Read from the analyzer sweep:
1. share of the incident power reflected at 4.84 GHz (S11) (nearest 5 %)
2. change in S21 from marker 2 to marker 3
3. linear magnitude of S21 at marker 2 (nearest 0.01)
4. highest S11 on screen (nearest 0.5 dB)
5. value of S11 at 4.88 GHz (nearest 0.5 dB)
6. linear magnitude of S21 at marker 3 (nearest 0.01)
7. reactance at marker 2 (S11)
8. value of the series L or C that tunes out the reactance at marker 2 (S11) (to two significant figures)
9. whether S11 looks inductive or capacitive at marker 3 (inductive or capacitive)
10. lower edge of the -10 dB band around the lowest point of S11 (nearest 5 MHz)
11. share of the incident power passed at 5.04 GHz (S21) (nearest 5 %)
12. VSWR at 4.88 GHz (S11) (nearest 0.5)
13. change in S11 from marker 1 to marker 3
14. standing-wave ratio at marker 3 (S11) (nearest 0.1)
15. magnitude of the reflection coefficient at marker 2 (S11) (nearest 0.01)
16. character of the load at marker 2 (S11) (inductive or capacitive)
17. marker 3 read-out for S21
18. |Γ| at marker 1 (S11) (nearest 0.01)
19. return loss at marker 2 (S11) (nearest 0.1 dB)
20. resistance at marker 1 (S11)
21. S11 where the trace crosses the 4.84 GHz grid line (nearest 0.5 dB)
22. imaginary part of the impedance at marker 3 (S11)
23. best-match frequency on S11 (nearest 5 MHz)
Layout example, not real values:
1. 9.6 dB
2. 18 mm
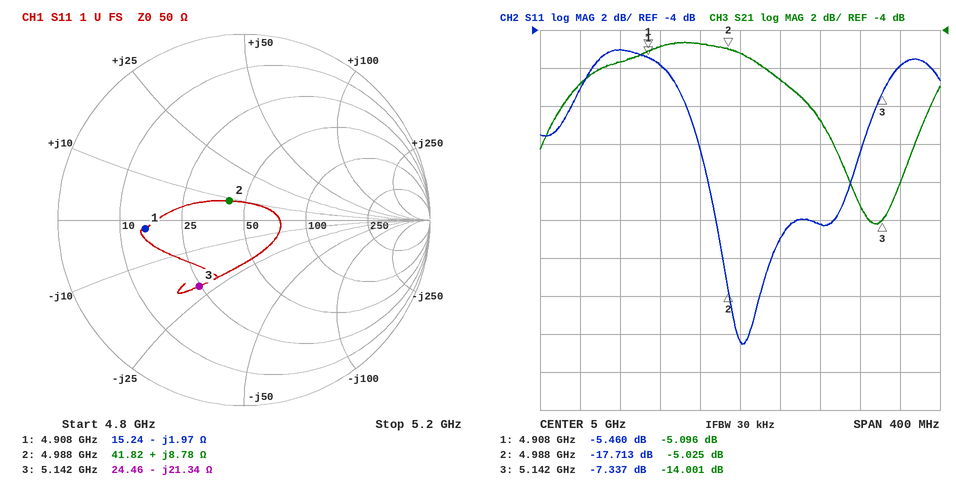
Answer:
1. 20 %
2. -8.976 dB
3. 0.56
4. -5.0 dB
5. -5.0 dB
6. 0.20
7. +8.78 Ω
8. 3.6 pF
9. capacitive
10. 4.960 GHz
11. 20 %
12. 3.5
13. -1.877 dB
14. 2.5
15. 0.13
16. inductive
17. -14.001 dB
18. 0.53
19. 17.7 dB
20. 15.24 Ω
21. -7.0 dB
22. -21.34 Ω
23. 5.000 GHz
